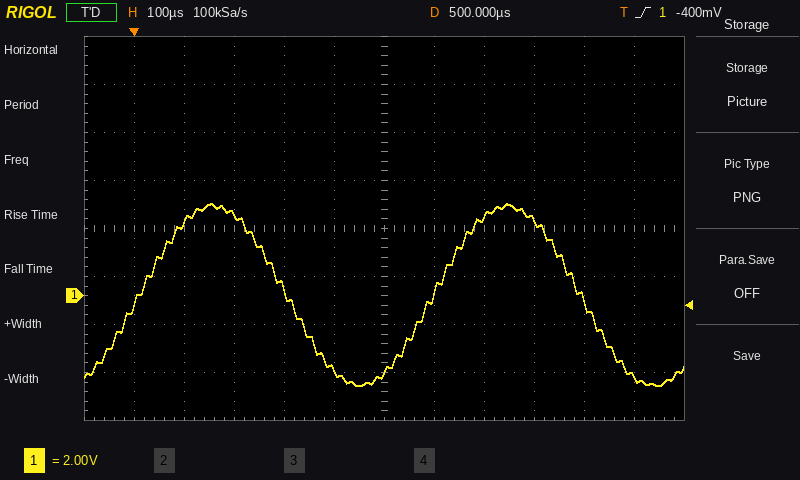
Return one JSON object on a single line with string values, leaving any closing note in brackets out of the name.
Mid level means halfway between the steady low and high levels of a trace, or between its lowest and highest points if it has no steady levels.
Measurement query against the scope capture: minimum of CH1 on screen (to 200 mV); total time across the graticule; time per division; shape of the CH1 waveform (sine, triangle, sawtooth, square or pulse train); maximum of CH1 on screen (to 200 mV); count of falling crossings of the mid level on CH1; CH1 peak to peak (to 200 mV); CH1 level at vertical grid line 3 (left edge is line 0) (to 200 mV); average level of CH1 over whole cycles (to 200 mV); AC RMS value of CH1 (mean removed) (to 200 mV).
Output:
{"minimum of CH1 on screen": "-3.8 V", "total time across the graticule": "1.2 ms", "time per division": "100 µs", "shape of the CH1 waveform": "sine", "maximum of CH1 on screen": "3.8 V", "count of falling crossings of the mid level on CH1": "2", "CH1 peak to peak": "7.6 V", "CH1 level at vertical grid line 3 (left edge is line 0)": "3.4 V", "average level of CH1 over whole cycles": "0.0 V", "AC RMS value of CH1 (mean removed)": "2.6 V"}
